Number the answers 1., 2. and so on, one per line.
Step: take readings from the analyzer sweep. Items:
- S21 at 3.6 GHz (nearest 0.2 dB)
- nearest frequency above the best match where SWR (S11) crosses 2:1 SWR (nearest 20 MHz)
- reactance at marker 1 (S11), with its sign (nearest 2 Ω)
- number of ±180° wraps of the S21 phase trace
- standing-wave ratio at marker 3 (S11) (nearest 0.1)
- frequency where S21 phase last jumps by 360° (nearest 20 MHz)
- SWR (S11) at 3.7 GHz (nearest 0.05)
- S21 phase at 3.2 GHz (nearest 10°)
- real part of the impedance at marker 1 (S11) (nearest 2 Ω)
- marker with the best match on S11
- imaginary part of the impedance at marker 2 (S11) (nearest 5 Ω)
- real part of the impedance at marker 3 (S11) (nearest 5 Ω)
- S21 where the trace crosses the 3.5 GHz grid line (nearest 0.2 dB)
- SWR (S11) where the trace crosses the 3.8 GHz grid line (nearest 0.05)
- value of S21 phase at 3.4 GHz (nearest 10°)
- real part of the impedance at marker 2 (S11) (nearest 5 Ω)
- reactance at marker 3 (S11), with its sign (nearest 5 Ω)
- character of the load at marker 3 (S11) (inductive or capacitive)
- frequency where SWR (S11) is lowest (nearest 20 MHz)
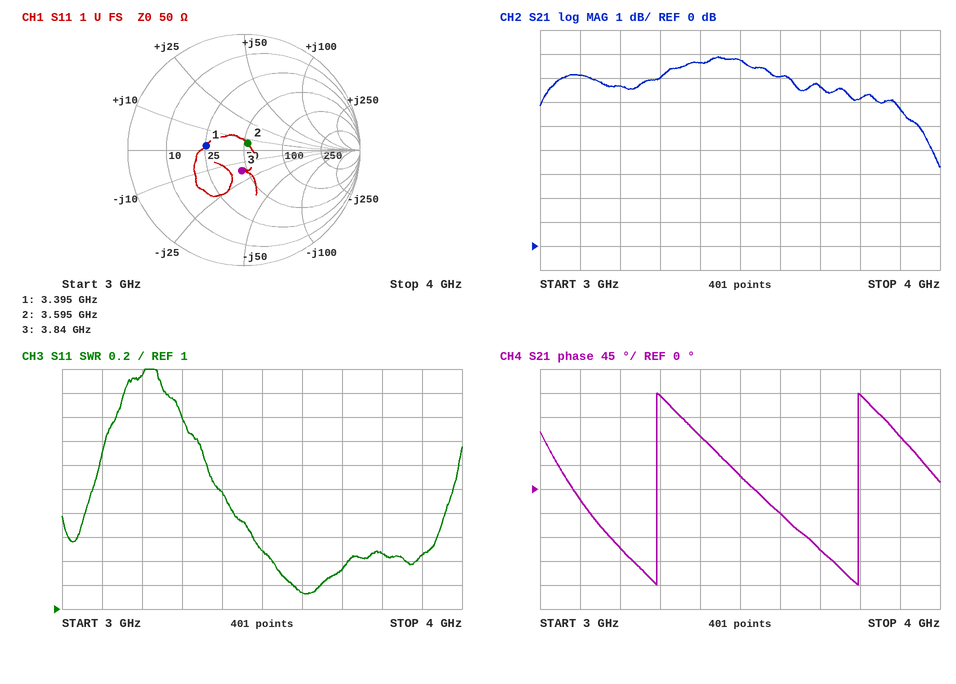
1. 7.0 dB
2. 3.98 GHz
3. +2 Ω
4. 2
5. 1.4
6. 3.80 GHz
7. 1.35
8. -110°
9. 26 Ω
10. marker 2
11. +5 Ω
12. 45 Ω
13. 7.8 dB
14. 1.45
15. 100°
16. 55 Ω
17. -15 Ω
18. capacitive
19. 3.60 GHz
